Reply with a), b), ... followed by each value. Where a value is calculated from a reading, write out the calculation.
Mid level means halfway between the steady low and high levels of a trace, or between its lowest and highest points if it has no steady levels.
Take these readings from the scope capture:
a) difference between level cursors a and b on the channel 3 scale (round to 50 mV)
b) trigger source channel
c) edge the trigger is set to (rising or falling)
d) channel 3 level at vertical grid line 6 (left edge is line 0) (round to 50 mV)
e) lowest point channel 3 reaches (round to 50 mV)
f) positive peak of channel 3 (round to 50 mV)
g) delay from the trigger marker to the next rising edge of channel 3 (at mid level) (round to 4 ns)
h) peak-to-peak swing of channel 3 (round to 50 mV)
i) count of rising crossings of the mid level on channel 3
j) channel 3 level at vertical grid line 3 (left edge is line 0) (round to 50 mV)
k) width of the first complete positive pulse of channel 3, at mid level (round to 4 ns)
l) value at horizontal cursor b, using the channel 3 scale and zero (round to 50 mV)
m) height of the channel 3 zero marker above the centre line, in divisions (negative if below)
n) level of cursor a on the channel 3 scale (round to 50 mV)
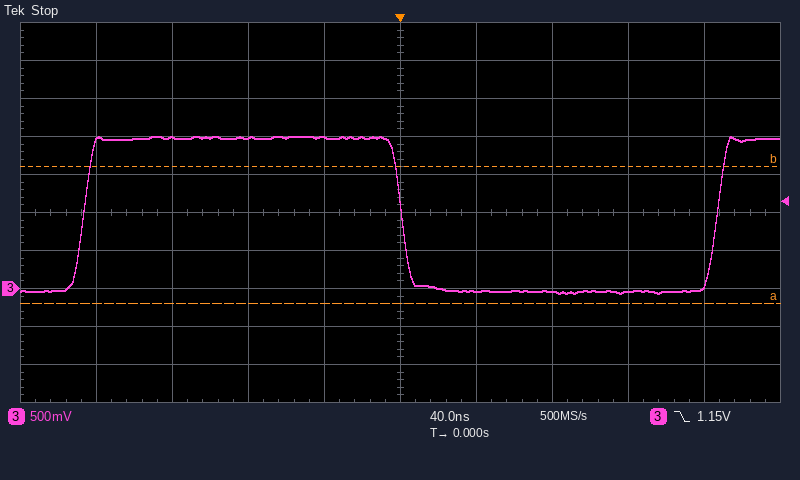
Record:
a) 1.80 V
b) channel 3
c) falling
d) -50 mV
e) -50 mV
f) 2.00 V
g) 168 ns
h) 2.00 V − (-50 mV) = 2.05 V
i) 2
j) 2.00 V
k) 168 ns
l) 1.60 V
m) -2.0 div
n) -200 mV
